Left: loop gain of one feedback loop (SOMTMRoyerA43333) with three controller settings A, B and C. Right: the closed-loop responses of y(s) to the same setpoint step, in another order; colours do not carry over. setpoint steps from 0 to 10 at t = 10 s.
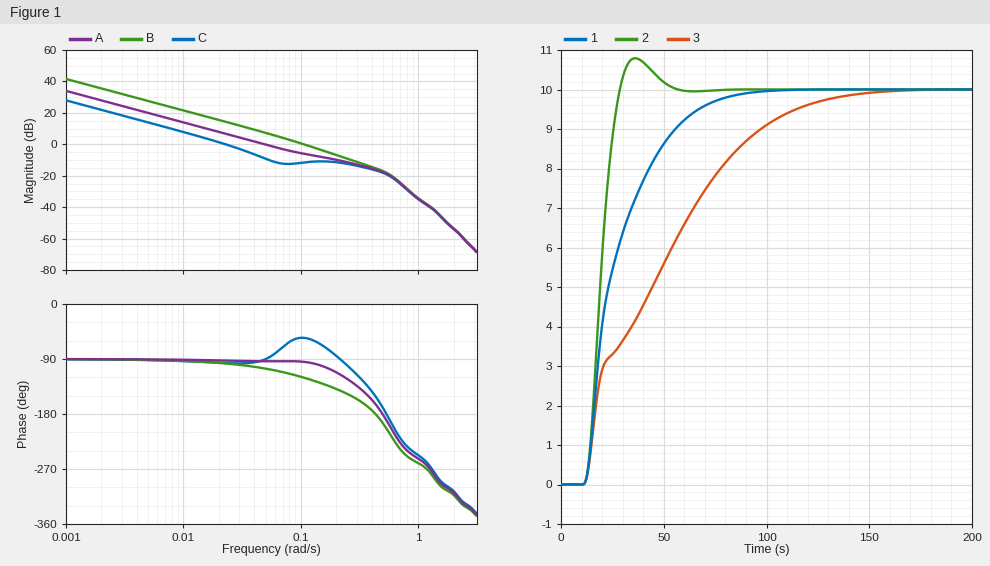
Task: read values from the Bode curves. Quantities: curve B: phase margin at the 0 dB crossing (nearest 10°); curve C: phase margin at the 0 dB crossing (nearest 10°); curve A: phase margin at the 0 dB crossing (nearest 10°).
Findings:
60°
80°
90°
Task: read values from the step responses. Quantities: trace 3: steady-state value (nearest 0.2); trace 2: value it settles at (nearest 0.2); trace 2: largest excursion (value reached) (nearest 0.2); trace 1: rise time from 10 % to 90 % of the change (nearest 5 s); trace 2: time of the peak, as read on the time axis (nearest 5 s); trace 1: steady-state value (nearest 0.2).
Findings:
10.0
10.0
10.8
40 s
35 s
10.0
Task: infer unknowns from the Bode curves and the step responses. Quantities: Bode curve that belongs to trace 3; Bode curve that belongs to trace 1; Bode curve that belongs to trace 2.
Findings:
C
A
B
